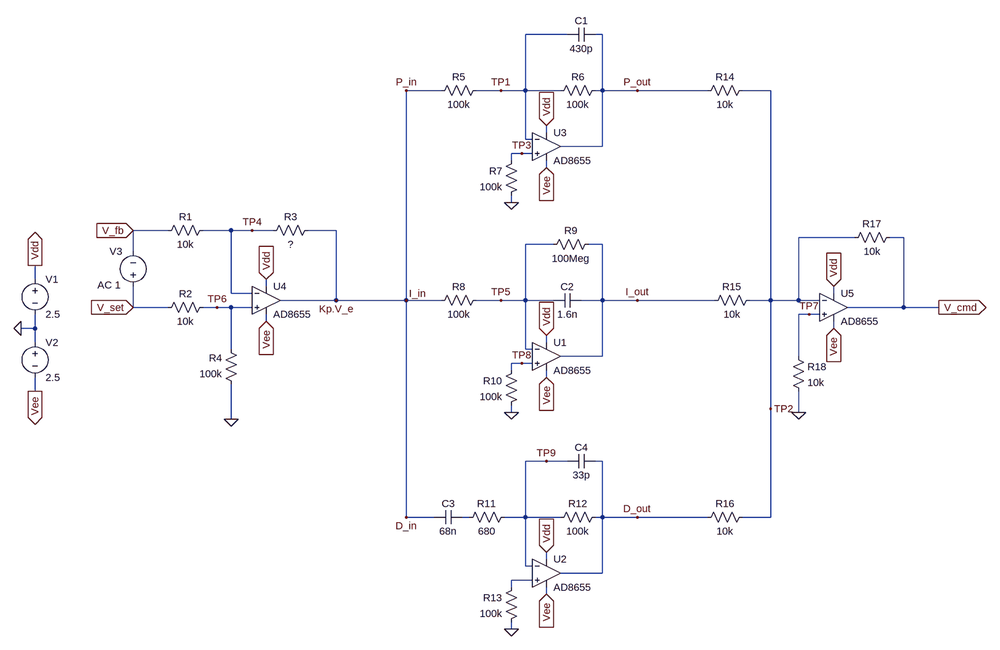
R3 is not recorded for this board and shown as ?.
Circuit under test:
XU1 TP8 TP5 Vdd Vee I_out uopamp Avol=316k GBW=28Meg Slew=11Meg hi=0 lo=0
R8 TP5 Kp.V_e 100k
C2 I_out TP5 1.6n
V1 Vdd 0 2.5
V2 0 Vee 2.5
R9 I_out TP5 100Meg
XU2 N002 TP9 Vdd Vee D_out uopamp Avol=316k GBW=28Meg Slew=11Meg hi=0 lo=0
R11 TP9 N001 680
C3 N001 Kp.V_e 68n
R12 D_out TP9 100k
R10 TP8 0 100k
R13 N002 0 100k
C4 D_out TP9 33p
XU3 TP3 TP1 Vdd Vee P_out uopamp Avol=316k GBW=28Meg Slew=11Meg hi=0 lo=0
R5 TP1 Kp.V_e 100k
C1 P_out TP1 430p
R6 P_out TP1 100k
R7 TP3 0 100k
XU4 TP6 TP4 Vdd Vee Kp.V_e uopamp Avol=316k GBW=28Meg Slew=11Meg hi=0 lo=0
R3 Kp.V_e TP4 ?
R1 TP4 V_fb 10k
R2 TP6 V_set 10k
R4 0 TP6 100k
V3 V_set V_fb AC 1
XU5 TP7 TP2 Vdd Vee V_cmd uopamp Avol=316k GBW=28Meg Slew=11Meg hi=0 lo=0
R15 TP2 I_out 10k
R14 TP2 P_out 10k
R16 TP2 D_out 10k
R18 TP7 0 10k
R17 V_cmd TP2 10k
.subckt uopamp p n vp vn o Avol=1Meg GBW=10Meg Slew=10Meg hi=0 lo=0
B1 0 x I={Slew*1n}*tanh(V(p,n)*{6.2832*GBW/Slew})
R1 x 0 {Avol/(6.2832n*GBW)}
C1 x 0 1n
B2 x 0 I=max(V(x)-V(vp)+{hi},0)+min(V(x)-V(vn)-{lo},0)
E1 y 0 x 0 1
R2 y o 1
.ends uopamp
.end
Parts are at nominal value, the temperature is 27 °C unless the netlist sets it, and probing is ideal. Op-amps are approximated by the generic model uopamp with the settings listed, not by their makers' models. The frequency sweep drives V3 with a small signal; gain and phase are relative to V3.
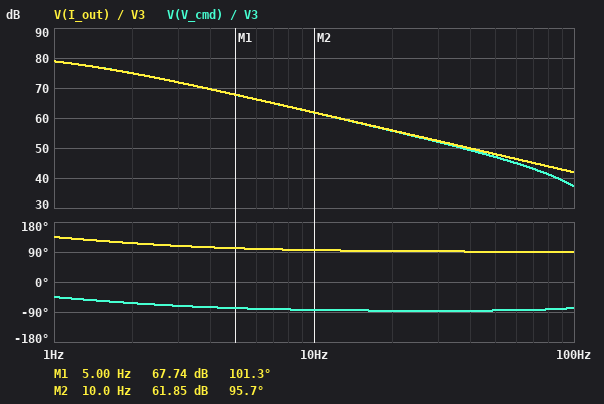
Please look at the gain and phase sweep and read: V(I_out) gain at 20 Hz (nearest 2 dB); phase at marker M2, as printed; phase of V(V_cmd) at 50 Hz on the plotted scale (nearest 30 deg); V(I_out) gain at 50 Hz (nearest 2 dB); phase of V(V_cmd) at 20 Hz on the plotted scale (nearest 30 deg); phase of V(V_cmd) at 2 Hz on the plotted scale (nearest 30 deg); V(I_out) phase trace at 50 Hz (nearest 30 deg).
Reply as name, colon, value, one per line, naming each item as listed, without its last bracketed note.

V(I_out) gain at 20 Hz: 56 dB
phase at marker M2, as printed: 95.7 deg
phase of V(V_cmd) at 50 Hz on the plotted scale: -90 deg
V(I_out) gain at 50 Hz: 48 dB
phase of V(V_cmd) at 20 Hz on the plotted scale: -90 deg
phase of V(V_cmd) at 2 Hz on the plotted scale: -60 deg
V(I_out) phase trace at 50 Hz: 90 deg
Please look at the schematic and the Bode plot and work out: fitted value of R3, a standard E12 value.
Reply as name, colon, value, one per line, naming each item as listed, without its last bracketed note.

fitted value of R3, a standard E12 value: 150 kΩ
